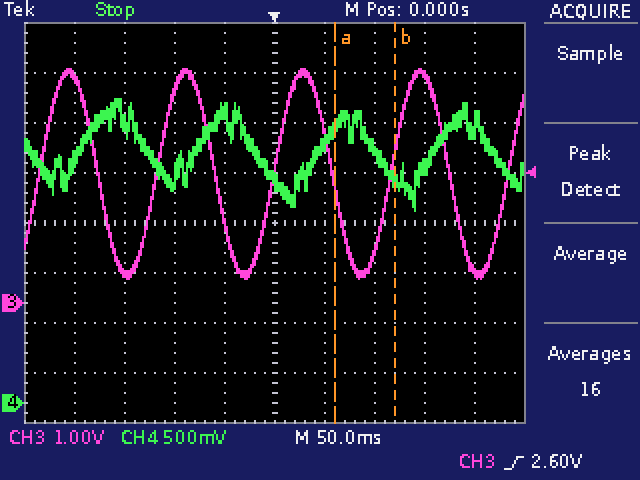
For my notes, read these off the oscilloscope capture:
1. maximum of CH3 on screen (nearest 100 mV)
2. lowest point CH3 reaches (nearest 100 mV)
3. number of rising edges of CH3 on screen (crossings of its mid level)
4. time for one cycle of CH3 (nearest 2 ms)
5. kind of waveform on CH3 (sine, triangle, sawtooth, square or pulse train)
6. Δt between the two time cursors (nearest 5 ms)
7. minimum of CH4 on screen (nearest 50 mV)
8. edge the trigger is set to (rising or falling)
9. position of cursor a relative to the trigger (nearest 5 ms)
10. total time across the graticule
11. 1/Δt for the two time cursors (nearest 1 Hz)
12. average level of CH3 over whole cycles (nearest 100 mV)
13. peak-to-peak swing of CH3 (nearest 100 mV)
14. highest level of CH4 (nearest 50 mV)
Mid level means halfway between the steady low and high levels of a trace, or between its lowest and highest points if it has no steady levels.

4.7 V
500 mV
5
118 ms
sine
60 ms
1.90 V
rising
+60 ms
500 ms
17 Hz
2.6 V
4.2 V
3.05 V
